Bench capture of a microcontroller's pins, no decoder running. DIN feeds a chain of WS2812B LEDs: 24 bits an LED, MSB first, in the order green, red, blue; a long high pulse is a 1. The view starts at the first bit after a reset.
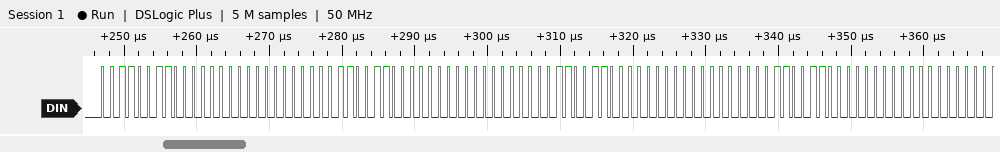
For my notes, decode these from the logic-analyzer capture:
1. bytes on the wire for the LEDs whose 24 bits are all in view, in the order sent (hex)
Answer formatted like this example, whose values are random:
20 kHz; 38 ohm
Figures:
33 00 00 33 00 00 33 00 00 33 00 00
